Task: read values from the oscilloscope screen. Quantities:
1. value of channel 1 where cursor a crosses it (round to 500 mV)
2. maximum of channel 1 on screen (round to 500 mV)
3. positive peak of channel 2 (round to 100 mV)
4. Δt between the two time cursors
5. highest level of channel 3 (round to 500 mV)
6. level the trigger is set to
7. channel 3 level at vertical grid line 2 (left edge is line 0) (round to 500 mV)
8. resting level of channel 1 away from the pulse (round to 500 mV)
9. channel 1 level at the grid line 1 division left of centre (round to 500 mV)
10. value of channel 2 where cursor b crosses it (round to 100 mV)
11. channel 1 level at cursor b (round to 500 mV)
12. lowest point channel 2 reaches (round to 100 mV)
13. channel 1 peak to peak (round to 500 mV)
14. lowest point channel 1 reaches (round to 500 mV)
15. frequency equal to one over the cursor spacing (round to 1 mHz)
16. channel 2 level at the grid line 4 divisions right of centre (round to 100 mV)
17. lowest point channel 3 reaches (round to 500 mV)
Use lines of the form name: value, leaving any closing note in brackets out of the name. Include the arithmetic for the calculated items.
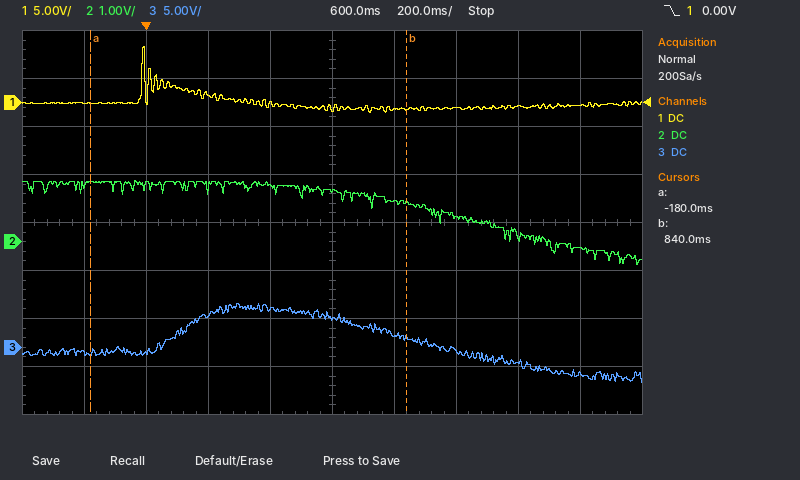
value of channel 1 where cursor a crosses it: 0.0 V
maximum of channel 1 on screen: 6.0 V
positive peak of channel 2: 1.3 V
Δt between the two time cursors: 840 ms − (-180 ms) = 1.02 s
highest level of channel 3: 4.5 V
level the trigger is set to: 0.00 V
channel 3 level at vertical grid line 2 (left edge is line 0): -500 mV
resting level of channel 1 away from the pulse: -500 mV
channel 1 level at the grid line 1 division left of centre: 0.0 V
value of channel 2 where cursor b crosses it: 800 mV
channel 1 level at cursor b: -500 mV
lowest point channel 2 reaches: -500 mV
channel 1 peak to peak: 6.0 V − (-1.0 V) = 7.0 V
lowest point channel 1 reaches: -1.0 V
frequency equal to one over the cursor spacing: 1 / 1.02 s ≈ 980 mHz
channel 2 level at the grid line 4 divisions right of centre: -100 mV
lowest point channel 3 reaches: -3.5 V
